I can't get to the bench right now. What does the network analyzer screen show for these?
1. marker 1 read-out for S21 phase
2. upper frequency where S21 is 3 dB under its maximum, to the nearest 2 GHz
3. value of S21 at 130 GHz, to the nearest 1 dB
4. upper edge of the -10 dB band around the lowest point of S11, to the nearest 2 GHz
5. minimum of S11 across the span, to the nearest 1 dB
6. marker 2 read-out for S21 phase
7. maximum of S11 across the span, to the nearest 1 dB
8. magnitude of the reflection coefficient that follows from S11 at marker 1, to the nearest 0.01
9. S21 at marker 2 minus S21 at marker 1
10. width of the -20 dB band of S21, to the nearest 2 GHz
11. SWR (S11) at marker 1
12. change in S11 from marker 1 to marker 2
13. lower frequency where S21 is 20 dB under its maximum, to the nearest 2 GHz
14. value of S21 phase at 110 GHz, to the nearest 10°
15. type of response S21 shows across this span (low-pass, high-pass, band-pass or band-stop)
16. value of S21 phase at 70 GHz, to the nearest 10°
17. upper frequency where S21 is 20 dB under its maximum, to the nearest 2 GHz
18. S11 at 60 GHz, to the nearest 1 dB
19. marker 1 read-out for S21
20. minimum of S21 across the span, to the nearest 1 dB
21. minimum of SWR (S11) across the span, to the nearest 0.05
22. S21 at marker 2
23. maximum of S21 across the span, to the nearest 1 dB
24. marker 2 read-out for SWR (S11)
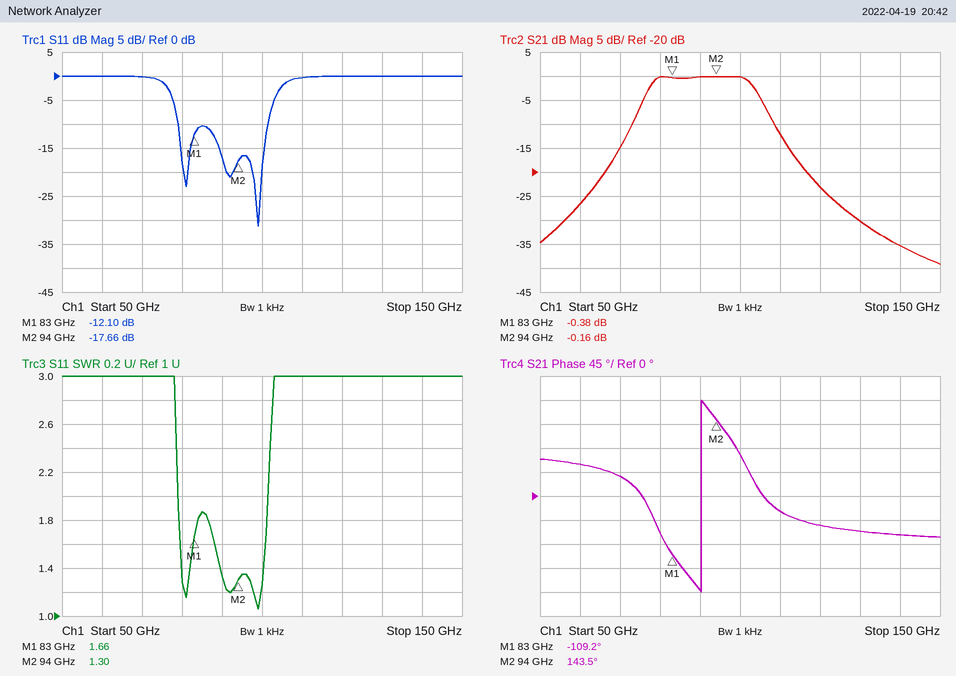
-109.2°
104 GHz
-30 dB
102 GHz
-31 dB
143.5°
0 dB
0.25
0.22 dB
50 GHz
1.66
-5.56 dB
66 GHz
-30°
band-pass
40°
116 GHz
0 dB
-0.38 dB
-39 dB
1.05
-0.16 dB
0 dB
1.30
